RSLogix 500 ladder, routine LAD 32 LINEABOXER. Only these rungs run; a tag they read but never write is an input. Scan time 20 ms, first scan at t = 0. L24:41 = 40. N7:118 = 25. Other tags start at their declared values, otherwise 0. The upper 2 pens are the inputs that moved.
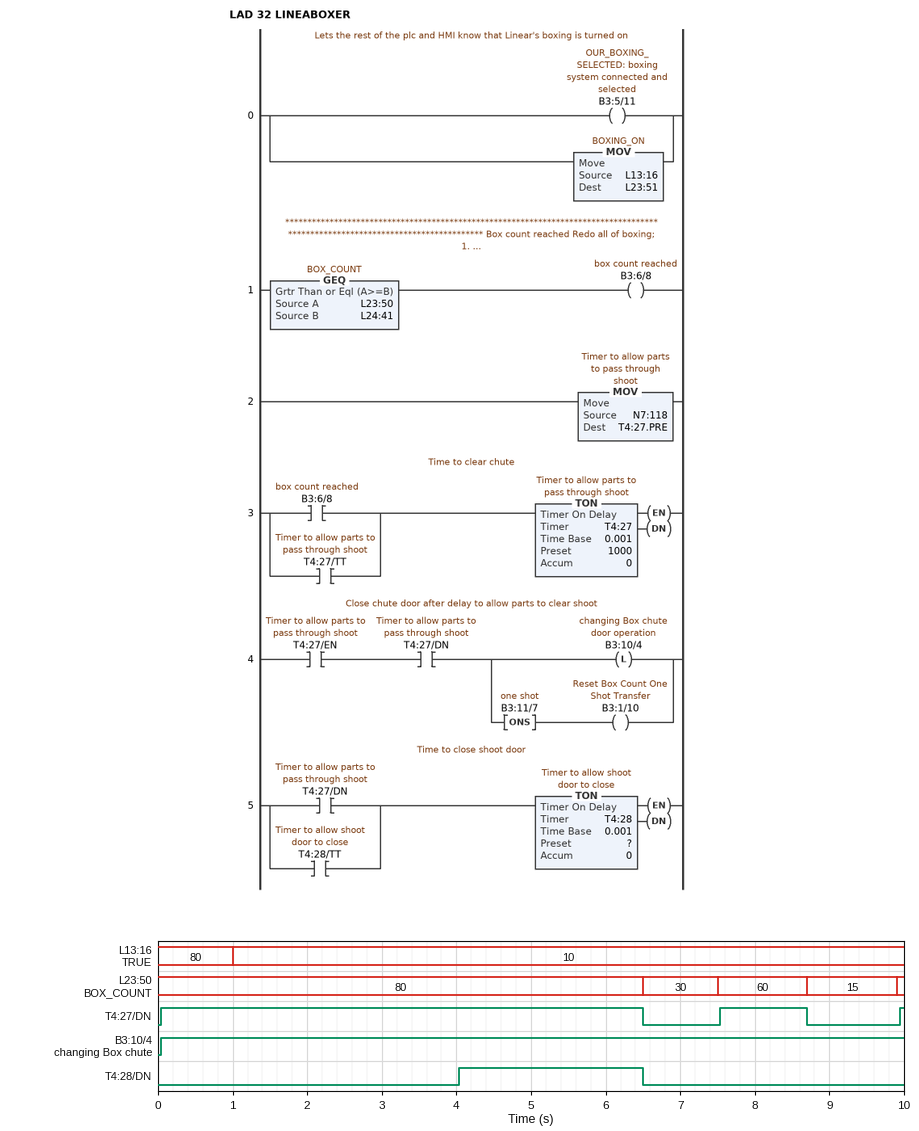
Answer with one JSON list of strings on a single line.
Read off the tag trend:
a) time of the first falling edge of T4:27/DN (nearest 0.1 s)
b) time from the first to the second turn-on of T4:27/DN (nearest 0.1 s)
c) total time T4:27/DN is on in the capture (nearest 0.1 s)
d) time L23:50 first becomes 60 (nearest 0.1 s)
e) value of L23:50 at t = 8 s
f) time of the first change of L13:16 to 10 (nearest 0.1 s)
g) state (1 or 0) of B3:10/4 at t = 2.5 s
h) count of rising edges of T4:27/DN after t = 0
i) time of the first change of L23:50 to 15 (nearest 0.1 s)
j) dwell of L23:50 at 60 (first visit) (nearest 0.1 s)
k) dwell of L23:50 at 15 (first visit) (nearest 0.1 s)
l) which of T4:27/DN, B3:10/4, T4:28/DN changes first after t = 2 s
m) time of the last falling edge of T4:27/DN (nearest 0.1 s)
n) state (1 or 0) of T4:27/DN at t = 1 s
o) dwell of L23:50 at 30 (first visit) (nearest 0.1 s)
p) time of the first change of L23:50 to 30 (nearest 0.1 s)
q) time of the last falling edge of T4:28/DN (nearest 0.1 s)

["6.5 s", "7.5 s", "7.7 s", "7.5 s", "60", "1.0 s", "1", "3", "8.7 s", "1.2 s", "1.2 s", "T4:28/DN", "8.7 s", "1", "1.0 s", "6.5 s", "6.5 s"]
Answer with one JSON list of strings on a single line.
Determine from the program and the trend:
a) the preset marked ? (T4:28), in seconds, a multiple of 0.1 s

["4.0 s"]
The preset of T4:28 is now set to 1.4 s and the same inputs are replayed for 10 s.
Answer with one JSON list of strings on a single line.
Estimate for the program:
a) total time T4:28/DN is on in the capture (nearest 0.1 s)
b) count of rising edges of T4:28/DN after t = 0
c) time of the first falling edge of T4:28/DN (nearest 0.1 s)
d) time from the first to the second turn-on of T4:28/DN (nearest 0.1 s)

["5.1 s", "2", "6.5 s", "7.5 s"]
